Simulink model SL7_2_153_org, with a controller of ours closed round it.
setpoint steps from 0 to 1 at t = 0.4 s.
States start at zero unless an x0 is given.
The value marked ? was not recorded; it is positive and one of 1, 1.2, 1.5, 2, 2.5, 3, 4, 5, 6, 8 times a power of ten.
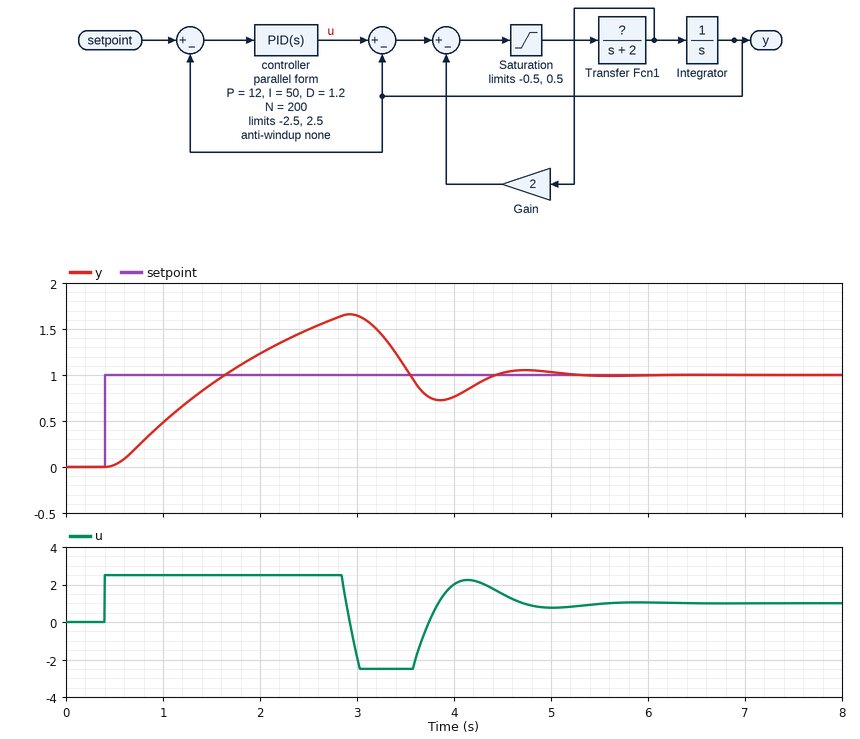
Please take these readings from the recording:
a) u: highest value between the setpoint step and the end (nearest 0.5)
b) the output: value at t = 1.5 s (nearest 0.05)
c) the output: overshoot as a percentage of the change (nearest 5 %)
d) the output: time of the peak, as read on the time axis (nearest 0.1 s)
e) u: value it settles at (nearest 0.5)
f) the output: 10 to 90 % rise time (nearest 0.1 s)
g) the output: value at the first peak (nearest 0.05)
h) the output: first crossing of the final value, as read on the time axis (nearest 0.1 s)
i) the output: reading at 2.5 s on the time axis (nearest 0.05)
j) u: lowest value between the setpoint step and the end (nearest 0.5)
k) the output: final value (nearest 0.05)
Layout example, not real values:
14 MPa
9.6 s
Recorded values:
2.5
0.90
65 %
2.9 s
1.0
0.9 s
1.65
1.6 s
1.50
-2.5
1.00
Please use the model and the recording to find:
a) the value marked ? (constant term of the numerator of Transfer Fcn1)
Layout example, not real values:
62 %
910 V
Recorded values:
10
